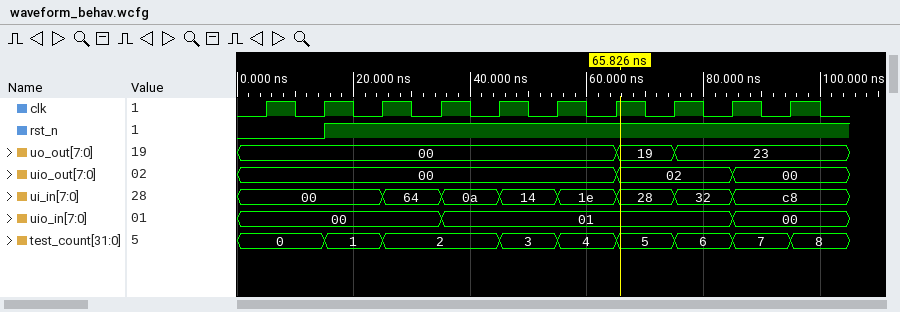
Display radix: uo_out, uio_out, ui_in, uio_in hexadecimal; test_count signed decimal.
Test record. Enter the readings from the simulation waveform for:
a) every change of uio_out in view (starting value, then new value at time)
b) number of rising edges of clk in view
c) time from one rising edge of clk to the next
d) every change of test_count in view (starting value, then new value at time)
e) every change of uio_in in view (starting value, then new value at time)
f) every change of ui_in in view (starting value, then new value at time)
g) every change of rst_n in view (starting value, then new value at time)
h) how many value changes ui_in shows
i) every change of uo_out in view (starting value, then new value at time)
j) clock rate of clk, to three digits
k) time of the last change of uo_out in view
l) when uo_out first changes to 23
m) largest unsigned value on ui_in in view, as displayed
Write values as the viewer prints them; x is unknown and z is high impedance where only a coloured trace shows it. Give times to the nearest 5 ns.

00, 02 at 65 ns, 00 at 85 ns
10
10 ns
0, 1 at 15 ns, 2 at 25 ns, 3 at 45 ns, 4 at 55 ns, 5 at 65 ns, 6 at 75 ns, 7 at 85 ns, 8 at 95 ns
00, 01 at 35 ns, 00 at 85 ns
00, 64 at 25 ns, 0a at 35 ns, 14 at 45 ns, 1e at 55 ns, 28 at 65 ns, 32 at 75 ns, c8 at 85 ns
0, 1 at 15 ns
7
00, 19 at 65 ns, 23 at 75 ns
100 MHz
75 ns
75 ns
c8
